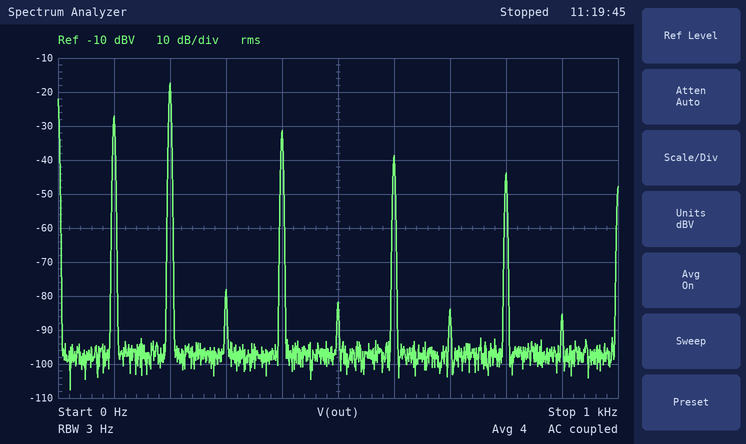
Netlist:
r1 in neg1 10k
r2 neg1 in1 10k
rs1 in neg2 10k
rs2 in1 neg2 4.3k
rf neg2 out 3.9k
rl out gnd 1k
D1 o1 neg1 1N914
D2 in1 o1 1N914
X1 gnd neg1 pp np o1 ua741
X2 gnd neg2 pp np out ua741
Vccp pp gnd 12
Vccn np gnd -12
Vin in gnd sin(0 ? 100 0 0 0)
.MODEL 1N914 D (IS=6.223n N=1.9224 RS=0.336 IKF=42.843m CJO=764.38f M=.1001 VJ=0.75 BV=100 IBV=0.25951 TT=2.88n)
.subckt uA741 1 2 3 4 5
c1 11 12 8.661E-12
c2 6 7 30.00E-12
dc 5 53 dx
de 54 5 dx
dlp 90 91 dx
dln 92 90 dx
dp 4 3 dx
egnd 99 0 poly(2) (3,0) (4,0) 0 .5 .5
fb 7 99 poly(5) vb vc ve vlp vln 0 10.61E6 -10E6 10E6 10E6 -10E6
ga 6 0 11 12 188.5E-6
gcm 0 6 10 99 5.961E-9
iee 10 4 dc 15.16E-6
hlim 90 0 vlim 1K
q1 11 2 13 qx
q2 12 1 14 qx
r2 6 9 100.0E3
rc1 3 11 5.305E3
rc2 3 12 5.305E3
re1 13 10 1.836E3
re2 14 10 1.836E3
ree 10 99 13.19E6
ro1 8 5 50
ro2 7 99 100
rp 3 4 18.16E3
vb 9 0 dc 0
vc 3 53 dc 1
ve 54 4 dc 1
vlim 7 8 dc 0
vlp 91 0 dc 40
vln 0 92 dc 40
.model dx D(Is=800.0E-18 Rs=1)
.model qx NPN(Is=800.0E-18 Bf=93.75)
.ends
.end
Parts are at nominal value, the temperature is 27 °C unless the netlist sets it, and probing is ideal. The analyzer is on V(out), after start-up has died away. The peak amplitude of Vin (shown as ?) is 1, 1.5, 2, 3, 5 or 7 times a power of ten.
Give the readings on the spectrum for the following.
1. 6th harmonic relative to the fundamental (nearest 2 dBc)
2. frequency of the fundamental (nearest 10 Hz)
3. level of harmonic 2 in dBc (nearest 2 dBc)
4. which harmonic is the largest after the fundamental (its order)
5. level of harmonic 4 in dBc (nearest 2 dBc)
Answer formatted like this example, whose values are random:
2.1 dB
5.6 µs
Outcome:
-12 dBc
100 Hz
10 dBc
2
-4 dBc
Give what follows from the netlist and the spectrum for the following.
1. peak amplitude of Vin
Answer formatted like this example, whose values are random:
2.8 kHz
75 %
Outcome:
1 V
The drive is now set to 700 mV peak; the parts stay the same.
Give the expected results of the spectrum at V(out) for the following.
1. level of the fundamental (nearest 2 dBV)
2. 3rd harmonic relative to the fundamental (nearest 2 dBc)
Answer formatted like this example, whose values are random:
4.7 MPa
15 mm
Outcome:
-30 dBV
-48 dBc
